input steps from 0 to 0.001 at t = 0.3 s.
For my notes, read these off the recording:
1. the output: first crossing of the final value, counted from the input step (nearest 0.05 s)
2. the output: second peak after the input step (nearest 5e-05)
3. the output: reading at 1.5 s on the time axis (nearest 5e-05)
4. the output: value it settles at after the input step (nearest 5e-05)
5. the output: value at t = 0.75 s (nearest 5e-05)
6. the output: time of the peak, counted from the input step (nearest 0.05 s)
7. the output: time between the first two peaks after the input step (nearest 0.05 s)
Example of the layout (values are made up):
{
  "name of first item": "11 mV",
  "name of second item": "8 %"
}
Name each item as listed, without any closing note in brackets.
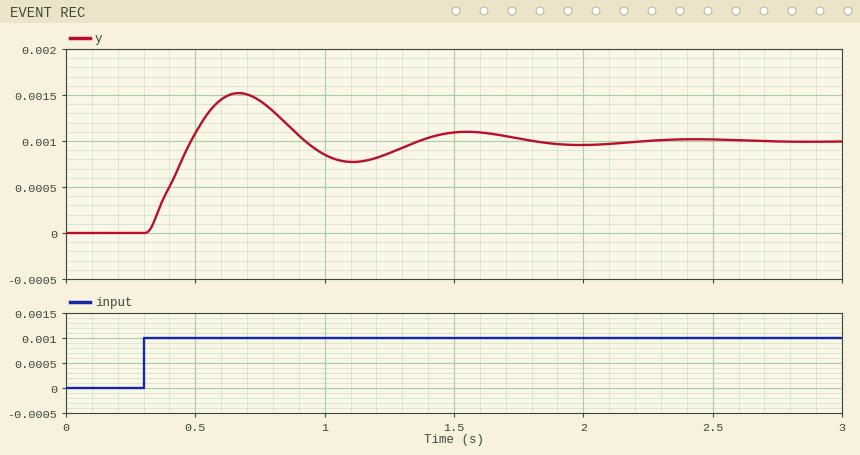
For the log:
{
  "the output: first crossing of the final value, counted from the input step": "0.20 s",
  "the output: second peak after the input step": "0.00110",
  "the output: reading at 1.5 s on the time axis": "0.00110",
  "the output: value it settles at after the input step": "0.00100",
  "the output: value at t = 0.75 s": "0.00145",
  "the output: time of the peak, counted from the input step": "0.35 s",
  "the output: time between the first two peaks after the input step": "0.90 s"
}
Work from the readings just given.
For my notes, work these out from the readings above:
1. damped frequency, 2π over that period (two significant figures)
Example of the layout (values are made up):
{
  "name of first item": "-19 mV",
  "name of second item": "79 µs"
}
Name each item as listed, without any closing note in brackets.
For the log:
{
  "damped frequency, 2π over that period": "7.0 rad/s"
}
